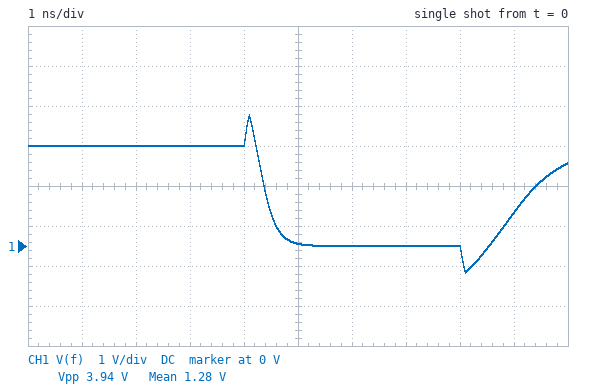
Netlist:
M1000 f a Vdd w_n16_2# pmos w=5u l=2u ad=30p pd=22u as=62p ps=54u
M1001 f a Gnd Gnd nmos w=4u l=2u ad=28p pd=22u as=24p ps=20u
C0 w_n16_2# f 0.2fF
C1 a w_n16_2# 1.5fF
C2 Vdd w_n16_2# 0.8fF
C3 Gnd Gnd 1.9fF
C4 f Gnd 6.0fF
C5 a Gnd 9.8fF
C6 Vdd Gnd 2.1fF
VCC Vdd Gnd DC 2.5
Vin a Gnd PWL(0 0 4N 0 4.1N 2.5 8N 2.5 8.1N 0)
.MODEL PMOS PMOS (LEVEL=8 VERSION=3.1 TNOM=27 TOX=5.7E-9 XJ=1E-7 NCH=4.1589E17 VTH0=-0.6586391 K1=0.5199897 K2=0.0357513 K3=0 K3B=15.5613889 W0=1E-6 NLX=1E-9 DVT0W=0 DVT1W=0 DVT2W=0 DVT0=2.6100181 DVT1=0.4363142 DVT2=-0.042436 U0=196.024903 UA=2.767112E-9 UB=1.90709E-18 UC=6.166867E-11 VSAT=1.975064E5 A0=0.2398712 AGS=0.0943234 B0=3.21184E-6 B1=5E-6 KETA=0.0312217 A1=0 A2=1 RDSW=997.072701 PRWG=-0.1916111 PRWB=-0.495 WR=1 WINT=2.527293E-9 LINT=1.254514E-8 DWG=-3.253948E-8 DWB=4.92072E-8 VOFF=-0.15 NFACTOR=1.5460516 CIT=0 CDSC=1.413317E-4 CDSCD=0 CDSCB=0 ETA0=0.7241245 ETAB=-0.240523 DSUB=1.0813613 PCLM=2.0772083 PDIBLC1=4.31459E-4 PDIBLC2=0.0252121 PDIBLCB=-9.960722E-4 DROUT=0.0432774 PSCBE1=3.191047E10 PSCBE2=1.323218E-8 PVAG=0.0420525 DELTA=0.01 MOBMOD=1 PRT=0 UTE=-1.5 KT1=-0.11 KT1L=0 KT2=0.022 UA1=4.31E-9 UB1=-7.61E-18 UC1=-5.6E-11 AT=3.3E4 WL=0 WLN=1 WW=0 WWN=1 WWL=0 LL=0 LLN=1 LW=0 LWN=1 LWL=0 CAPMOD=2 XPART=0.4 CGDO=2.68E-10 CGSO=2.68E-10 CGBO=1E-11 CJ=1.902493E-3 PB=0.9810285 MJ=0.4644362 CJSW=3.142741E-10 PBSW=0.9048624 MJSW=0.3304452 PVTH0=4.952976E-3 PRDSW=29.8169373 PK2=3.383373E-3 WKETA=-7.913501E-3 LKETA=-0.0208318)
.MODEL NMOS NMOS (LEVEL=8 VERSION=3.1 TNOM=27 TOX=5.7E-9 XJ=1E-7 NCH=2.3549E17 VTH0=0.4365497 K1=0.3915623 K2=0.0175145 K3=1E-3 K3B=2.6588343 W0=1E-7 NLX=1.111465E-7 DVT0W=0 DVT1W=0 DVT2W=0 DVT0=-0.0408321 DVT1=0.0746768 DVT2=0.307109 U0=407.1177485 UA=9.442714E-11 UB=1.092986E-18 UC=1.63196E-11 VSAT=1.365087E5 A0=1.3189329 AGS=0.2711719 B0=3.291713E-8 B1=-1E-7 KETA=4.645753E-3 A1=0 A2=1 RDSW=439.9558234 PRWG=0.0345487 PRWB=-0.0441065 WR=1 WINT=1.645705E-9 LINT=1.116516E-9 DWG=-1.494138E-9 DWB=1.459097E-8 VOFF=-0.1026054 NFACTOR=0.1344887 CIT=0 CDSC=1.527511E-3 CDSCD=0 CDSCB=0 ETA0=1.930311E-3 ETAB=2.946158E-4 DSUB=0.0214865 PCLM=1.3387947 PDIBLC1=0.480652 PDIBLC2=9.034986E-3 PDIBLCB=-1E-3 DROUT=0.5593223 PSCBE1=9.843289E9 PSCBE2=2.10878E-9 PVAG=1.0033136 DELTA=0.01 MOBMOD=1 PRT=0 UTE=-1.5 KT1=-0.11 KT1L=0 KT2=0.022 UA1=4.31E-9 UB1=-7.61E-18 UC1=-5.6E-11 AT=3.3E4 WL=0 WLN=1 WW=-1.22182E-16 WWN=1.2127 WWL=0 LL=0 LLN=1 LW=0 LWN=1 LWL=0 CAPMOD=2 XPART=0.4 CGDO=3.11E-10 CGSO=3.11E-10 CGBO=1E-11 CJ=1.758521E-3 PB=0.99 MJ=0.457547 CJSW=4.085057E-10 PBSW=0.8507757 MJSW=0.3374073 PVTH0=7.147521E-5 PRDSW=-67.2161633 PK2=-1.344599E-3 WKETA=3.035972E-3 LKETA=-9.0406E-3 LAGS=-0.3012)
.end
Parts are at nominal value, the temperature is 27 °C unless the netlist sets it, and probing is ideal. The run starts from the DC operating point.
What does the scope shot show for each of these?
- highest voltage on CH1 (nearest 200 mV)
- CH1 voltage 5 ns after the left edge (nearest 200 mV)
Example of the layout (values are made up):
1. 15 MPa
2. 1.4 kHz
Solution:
1. 3.2 V
2. 0 V
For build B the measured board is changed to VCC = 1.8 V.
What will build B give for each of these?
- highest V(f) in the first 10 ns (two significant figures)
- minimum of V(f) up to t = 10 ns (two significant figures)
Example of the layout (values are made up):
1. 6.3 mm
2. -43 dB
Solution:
1. 2.4 V
2. -650 mV
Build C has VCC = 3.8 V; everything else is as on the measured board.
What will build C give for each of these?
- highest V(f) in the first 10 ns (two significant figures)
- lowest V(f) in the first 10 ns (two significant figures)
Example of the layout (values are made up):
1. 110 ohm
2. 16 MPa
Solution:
1. 4.6 V
2. -600 mV
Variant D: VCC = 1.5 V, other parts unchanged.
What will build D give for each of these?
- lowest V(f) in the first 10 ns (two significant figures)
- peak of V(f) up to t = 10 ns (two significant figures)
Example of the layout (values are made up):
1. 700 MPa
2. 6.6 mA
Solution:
1. -640 mV
2. 2.1 V
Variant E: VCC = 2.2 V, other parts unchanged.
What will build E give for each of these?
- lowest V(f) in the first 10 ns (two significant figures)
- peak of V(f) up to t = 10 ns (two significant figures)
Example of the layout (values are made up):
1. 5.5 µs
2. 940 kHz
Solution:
1. -670 mV
2. 2.9 V
